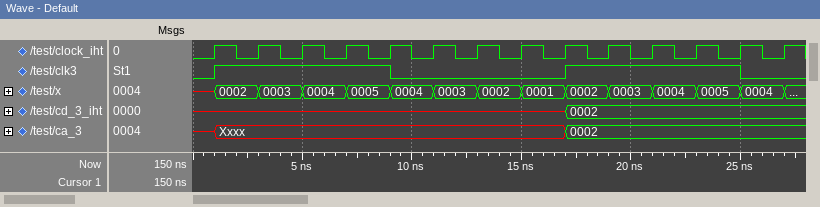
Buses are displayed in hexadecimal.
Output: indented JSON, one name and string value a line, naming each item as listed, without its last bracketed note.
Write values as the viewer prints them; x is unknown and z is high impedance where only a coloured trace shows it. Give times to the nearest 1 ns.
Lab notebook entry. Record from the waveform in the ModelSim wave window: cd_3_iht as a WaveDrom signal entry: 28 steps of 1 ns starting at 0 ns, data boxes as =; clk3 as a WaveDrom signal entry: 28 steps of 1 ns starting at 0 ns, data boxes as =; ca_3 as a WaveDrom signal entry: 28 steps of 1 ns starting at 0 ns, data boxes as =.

{
  "cd_3_iht as a WaveDrom signal entry: 28 steps of 1 ns starting at 0 ns, data boxes as =": "{name: 'cd_3_iht', wave: 'x................=..........', data: '0002'}",
  "clk3 as a WaveDrom signal entry: 28 steps of 1 ns starting at 0 ns, data boxes as =": "{name: 'clk3', wave: '01.......0.......1.......0..'}",
  "ca_3 as a WaveDrom signal entry: 28 steps of 1 ns starting at 0 ns, data boxes as =": "{name: 'ca_3', wave: 'x=...............=..........', data: 'Xxxx 0002'}"
}
